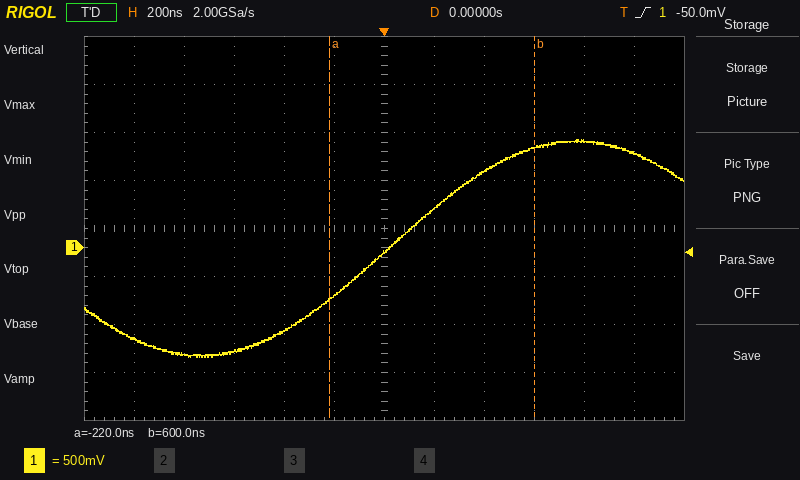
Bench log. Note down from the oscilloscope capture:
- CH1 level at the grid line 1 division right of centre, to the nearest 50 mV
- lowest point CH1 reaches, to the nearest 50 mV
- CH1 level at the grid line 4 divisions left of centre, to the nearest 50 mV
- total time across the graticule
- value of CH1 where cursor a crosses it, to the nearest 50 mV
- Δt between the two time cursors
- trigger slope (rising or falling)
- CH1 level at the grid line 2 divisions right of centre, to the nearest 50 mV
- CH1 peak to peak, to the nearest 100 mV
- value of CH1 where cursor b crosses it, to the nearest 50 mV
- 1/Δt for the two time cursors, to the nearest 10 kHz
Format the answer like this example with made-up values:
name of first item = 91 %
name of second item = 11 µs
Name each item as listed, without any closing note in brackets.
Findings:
CH1 level at the grid line 1 division right of centre, to the nearest 50 mV = 400 mV
lowest point CH1 reaches, to the nearest 50 mV = -1.15 V
CH1 level at the grid line 4 divisions left of centre, to the nearest 50 mV = -1.10 V
total time across the graticule = 2.4 µs
value of CH1 where cursor a crosses it, to the nearest 50 mV = -550 mV
Δt between the two time cursors = 820 ns
trigger slope = rising
CH1 level at the grid line 2 divisions right of centre, to the nearest 50 mV = 800 mV
CH1 peak to peak, to the nearest 100 mV = 2.30 V
value of CH1 where cursor b crosses it, to the nearest 50 mV = 1.05 V
1/Δt for the two time cursors, to the nearest 10 kHz = 1.22 MHz
